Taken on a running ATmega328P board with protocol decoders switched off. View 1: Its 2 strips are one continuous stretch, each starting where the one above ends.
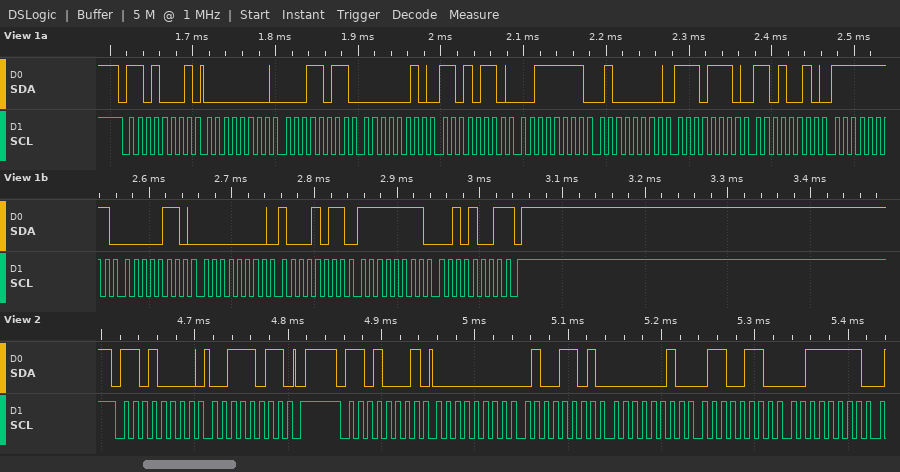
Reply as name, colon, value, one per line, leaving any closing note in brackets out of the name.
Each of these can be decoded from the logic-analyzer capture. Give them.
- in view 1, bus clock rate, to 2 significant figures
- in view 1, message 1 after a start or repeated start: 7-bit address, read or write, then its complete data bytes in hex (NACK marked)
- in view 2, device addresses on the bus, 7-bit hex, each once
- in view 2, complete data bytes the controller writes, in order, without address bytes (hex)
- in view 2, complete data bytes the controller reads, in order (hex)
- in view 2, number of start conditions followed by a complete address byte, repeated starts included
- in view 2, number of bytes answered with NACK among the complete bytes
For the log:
in view 1, bus clock rate, to 2 significant figures: 100 kHz
in view 1, message 1 after a start or repeated start: 7-bit address, read or write, then its complete data bytes in hex: 0x68 read: 00 1B 02 D6 3F 40 EE D2 FF 06 00 8B FF 29 NACK
in view 2, device addresses on the bus, 7-bit hex, each once: 0x68
in view 2, complete data bytes the controller writes, in order, without address bytes: 3B
in view 2, complete data bytes the controller reads, in order: 00 4D 02 66 3F
in view 2, number of start conditions followed by a complete address byte, repeated starts included: 2
in view 2, number of bytes answered with NACK among the complete bytes: 0
